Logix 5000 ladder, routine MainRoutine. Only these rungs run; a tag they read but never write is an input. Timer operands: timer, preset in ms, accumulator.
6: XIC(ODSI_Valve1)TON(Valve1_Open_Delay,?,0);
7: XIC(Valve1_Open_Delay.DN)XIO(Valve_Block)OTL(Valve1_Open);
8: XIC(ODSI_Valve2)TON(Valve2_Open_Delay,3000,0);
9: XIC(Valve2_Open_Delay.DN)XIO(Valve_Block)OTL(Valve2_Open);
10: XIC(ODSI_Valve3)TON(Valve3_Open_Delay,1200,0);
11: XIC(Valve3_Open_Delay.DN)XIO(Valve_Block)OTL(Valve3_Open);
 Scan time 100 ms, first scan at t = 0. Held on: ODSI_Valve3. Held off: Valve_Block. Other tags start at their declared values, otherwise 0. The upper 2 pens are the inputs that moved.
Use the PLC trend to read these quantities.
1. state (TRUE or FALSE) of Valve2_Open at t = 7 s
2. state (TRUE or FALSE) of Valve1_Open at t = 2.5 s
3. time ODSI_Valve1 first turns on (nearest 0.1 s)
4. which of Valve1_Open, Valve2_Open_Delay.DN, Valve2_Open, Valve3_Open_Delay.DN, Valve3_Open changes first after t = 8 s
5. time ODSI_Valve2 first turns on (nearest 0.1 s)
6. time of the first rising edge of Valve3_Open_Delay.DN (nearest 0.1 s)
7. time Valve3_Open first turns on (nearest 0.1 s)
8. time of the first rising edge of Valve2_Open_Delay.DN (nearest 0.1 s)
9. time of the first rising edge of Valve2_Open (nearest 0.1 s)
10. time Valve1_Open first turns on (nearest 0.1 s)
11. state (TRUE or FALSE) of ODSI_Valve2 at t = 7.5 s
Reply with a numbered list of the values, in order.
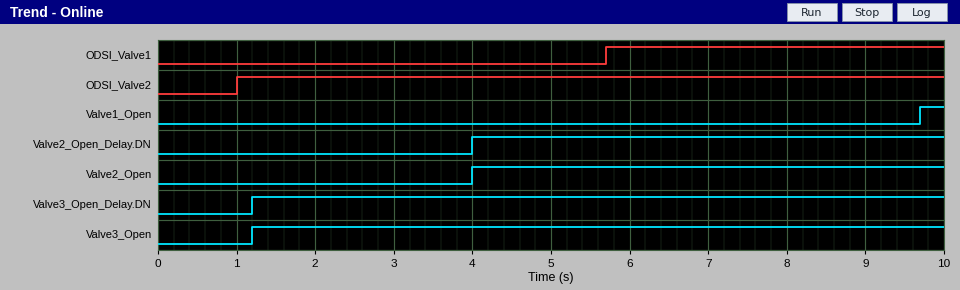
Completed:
1. TRUE
2. FALSE
3. 5.7 s
4. Valve1_Open
5. 1.0 s
6. 1.2 s
7. 1.2 s
8. 4.0 s
9. 4.0 s
10. 9.7 s
11. TRUE
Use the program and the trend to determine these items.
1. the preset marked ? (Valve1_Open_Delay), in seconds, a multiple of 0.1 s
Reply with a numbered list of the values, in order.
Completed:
1. 4.0 s
